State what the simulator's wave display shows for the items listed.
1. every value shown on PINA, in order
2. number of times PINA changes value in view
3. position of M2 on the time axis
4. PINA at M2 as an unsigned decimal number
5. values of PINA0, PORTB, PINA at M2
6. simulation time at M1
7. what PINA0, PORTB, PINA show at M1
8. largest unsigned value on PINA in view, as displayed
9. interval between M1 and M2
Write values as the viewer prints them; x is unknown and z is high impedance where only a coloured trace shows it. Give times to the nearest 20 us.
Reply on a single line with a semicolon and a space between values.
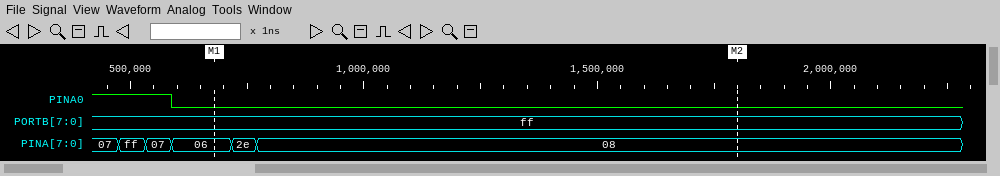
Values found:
07, ff, 07, 06, 2e, 08; 5; 1800 us; 8; PINA0=0, PORTB=ff, PINA=08; 680 us; PINA0=0, PORTB=ff, PINA=06; ff; 1120 us
